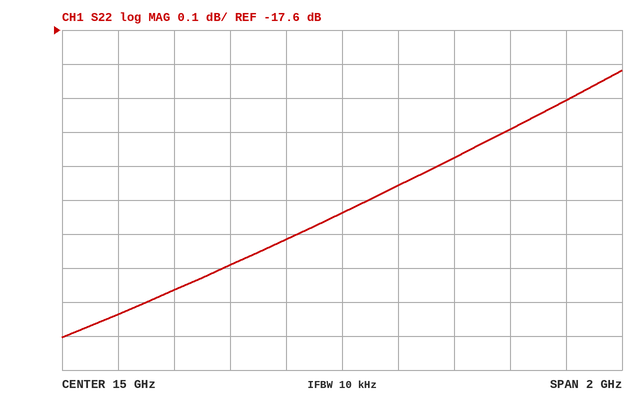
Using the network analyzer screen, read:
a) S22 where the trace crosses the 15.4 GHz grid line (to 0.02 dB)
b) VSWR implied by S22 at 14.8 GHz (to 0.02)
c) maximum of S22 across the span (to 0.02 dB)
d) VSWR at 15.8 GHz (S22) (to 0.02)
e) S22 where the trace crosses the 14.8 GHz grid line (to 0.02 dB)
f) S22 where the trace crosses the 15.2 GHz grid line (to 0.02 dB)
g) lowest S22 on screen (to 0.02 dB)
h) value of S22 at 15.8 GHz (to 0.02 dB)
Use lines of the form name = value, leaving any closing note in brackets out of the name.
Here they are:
S22 where the trace crosses the 15.4 GHz grid line = -17.98 dB
VSWR implied by S22 at 14.8 GHz = 1.28
maximum of S22 across the span = -17.72 dB
VSWR at 15.8 GHz (S22) = 1.30
S22 where the trace crosses the 14.8 GHz grid line = -18.22 dB
S22 where the trace crosses the 15.2 GHz grid line = -18.06 dB
lowest S22 on screen = -18.50 dB
value of S22 at 15.8 GHz = -17.80 dB
